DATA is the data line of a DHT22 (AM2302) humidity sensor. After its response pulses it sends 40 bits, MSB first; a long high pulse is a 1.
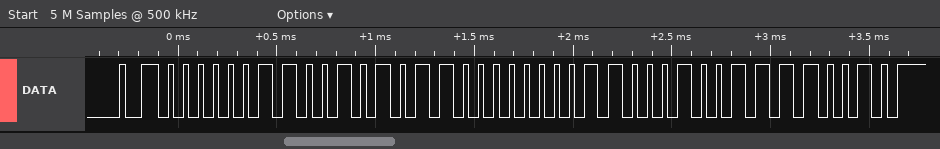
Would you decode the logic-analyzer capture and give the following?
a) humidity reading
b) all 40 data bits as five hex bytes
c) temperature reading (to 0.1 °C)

81.1 %
03 2B 00 C4 F2
19.6 °C
